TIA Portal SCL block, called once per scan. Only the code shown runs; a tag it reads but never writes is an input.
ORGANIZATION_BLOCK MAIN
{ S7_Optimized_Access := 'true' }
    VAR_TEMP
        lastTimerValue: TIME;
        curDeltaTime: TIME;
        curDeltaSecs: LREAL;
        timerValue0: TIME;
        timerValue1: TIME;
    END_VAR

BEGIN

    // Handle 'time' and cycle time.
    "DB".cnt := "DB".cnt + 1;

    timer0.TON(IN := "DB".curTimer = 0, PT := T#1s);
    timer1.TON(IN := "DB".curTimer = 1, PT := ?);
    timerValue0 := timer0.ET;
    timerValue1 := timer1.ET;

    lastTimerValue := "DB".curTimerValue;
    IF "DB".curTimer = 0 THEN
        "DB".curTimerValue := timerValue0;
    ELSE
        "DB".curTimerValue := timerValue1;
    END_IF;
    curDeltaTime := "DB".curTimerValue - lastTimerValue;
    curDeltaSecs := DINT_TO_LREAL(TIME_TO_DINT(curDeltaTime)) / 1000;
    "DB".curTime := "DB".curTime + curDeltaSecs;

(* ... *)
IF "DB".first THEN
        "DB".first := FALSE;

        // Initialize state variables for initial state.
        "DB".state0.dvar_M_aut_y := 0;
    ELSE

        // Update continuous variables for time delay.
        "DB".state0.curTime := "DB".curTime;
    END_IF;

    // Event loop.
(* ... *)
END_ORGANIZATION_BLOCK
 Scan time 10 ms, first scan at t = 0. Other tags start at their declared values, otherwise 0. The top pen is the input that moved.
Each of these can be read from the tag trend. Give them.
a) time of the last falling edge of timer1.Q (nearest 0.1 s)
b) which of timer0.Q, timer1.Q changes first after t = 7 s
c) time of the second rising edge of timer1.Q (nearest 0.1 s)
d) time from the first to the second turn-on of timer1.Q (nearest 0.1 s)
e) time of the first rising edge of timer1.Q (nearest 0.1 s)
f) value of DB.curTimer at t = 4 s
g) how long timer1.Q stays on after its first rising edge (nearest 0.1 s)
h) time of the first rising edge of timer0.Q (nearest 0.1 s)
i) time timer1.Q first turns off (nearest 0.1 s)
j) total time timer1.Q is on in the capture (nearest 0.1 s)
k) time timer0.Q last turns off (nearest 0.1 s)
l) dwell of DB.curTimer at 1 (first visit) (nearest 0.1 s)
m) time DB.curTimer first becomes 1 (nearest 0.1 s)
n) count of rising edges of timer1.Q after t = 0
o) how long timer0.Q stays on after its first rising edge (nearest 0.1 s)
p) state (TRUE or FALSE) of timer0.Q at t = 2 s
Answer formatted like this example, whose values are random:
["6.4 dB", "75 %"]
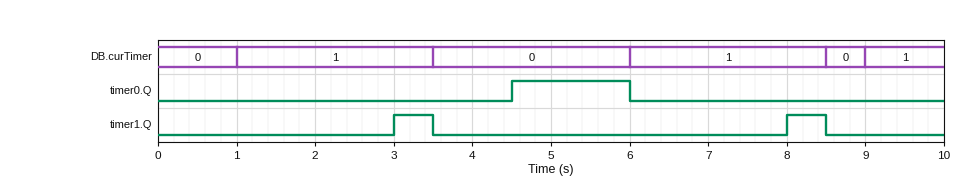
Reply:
["8.5 s", "timer1.Q", "8.0 s", "5.0 s", "3.0 s", "0", "0.5 s", "4.5 s", "3.5 s", "1.0 s", "6.0 s", "2.5 s", "1.0 s", "2", "1.5 s", "FALSE"]
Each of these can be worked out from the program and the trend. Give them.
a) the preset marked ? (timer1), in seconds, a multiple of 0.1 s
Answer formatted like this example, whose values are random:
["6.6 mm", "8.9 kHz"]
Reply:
["2.0 s"]
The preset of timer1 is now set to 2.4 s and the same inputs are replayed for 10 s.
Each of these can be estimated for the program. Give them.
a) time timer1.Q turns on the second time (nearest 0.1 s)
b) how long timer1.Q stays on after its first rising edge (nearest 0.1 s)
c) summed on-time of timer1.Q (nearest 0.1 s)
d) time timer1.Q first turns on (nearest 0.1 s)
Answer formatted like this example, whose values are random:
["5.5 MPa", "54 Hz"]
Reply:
["8.4 s", "0.1 s", "0.2 s", "3.4 s"]
